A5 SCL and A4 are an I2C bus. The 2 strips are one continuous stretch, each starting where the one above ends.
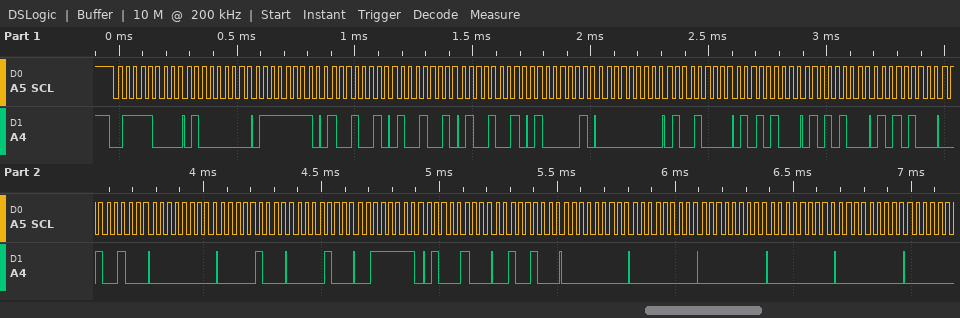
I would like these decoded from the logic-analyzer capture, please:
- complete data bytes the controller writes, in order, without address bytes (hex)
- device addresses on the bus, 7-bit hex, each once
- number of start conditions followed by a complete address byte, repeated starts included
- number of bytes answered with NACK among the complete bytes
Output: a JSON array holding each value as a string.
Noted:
["40 7F 49 49 49 41 00 48 54 54 54 24 00 04 04 3F 44 24 00 00 00 00 00", "0x3C", "1", "0"]
